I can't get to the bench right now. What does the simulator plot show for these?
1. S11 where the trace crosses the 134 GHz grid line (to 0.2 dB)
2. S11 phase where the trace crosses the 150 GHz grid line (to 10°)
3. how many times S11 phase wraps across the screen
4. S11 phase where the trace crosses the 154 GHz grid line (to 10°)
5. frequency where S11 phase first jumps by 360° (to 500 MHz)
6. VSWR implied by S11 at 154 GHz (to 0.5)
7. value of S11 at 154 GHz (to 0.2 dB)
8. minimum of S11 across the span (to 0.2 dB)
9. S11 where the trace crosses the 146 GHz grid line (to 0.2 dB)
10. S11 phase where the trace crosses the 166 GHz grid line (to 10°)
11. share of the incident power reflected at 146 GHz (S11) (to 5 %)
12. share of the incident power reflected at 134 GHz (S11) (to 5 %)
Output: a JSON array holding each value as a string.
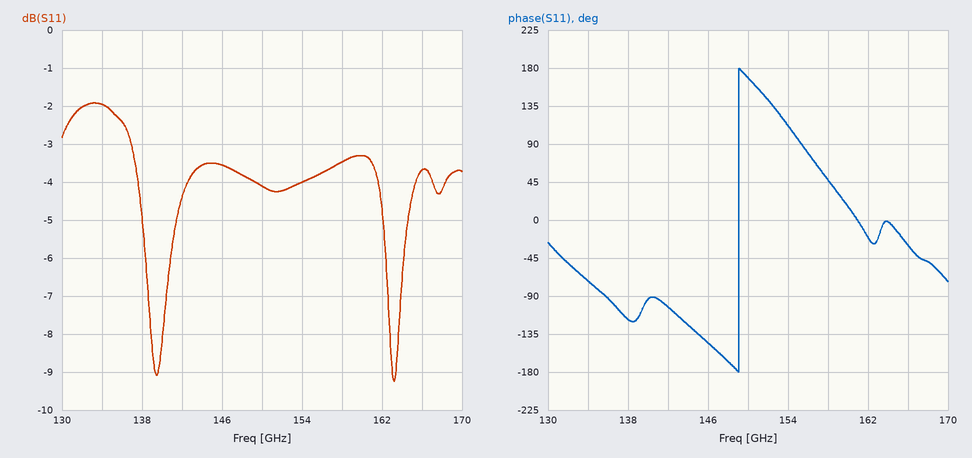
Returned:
["-2.0 dB", "170°", "1", "110°", "149.0 GHz", "4.5", "-4.0 dB", "-9.2 dB", "-3.6 dB", "-30°", "45 %", "65 %"]
